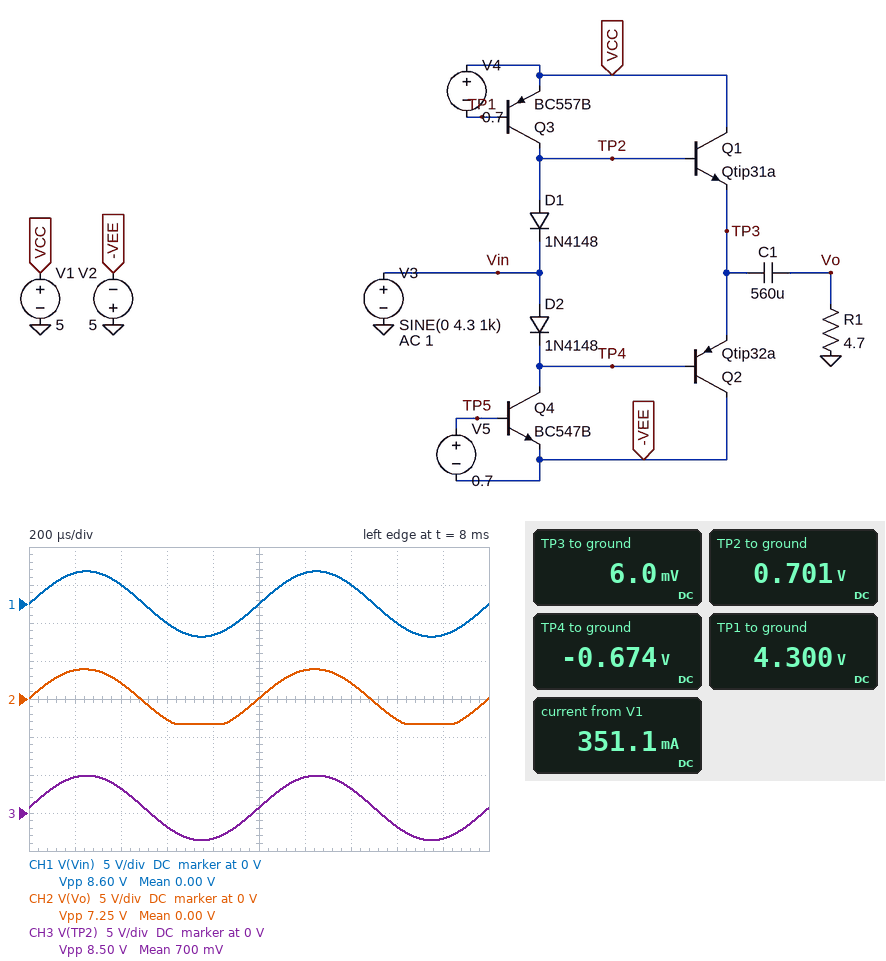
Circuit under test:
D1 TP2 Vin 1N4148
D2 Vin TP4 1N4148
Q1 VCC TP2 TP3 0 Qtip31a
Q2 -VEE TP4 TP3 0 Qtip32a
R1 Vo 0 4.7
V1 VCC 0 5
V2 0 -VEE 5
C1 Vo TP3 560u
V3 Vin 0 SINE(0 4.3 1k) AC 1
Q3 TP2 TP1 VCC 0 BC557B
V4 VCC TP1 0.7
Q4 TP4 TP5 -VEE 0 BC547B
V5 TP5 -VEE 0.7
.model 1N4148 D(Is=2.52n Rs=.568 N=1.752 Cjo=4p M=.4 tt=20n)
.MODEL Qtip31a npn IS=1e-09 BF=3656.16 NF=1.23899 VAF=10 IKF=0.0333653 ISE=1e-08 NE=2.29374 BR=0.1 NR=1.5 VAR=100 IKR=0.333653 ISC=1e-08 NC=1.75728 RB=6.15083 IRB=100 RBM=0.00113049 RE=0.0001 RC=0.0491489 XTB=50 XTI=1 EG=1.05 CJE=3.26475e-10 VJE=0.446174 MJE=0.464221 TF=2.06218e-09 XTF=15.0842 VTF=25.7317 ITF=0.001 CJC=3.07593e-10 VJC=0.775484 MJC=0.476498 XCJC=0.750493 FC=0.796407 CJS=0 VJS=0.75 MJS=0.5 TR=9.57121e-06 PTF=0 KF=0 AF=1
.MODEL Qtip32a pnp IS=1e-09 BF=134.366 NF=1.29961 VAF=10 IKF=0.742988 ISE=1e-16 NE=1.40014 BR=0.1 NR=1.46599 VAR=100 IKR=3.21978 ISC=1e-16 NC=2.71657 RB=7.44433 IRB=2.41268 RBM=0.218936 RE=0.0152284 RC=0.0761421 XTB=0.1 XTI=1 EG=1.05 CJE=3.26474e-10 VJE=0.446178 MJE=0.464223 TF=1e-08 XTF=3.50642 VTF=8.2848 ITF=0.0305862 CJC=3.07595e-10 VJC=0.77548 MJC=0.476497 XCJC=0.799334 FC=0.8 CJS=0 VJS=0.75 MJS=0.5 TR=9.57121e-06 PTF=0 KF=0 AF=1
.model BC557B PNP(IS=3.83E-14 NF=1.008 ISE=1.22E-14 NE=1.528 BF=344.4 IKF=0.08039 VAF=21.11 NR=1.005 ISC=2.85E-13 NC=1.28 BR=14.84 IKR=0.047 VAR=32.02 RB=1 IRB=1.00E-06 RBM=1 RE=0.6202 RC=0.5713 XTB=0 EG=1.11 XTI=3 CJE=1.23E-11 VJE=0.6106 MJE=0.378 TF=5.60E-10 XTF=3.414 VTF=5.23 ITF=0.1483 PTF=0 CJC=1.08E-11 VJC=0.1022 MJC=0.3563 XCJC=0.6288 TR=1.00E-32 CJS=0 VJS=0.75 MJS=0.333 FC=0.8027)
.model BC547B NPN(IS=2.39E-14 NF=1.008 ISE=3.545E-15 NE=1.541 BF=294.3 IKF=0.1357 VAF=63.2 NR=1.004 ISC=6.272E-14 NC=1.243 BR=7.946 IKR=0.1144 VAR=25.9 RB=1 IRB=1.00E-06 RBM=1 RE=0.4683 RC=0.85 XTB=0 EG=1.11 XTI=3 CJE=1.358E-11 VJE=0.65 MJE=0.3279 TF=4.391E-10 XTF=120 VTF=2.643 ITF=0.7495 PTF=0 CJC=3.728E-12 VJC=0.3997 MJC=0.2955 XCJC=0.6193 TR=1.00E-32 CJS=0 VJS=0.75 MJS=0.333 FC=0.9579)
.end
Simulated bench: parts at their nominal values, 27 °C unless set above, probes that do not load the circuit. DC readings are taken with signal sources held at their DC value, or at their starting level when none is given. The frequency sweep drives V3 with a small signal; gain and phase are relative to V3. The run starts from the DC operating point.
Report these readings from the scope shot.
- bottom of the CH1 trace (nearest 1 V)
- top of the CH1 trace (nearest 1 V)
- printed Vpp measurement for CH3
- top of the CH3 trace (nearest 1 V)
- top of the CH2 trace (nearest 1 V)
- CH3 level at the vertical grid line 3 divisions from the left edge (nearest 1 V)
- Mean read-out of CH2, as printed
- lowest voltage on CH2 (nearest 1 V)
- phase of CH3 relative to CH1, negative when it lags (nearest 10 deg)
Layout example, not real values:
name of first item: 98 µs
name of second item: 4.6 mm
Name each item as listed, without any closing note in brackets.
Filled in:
bottom of the CH1 trace: -4 V
top of the CH1 trace: 4 V
printed Vpp measurement for CH3: 8.50 V
top of the CH3 trace: 5 V
top of the CH2 trace: 4 V
CH3 level at the vertical grid line 3 divisions from the left edge: -2 V
Mean read-out of CH2, as printed: 0.00 V
lowest voltage on CH2: -3 V
phase of CH3 relative to CH1, negative when it lags: 0 deg
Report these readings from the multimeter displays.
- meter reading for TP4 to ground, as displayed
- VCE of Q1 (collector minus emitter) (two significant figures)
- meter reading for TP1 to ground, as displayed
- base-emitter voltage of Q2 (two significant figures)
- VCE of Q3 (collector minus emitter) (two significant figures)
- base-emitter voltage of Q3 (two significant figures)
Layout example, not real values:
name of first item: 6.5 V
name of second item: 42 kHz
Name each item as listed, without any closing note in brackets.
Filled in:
meter reading for TP4 to ground, as displayed: -0.674 V
VCE of Q1 (collector minus emitter): 5.0 V
meter reading for TP1 to ground, as displayed: 4.300 V
base-emitter voltage of Q2: -680 mV
VCE of Q3 (collector minus emitter): -4.3 V
base-emitter voltage of Q3: -700 mV
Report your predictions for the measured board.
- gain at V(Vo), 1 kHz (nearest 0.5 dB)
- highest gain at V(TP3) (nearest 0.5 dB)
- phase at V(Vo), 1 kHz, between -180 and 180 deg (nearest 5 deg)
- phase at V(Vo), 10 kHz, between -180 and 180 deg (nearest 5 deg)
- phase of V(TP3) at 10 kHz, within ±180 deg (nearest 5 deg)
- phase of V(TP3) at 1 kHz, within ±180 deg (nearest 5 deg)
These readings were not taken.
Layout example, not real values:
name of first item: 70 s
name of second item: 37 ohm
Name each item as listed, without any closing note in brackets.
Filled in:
gain at V(Vo), 1 kHz: -0.5 dB
highest gain at V(TP3): 0 dB
phase at V(Vo), 1 kHz, between -180 and 180 deg: 5 deg
phase at V(Vo), 10 kHz, between -180 and 180 deg: 0 deg
phase of V(TP3) at 10 kHz, within ±180 deg: 0 deg
phase of V(TP3) at 1 kHz, within ±180 deg: 0 deg
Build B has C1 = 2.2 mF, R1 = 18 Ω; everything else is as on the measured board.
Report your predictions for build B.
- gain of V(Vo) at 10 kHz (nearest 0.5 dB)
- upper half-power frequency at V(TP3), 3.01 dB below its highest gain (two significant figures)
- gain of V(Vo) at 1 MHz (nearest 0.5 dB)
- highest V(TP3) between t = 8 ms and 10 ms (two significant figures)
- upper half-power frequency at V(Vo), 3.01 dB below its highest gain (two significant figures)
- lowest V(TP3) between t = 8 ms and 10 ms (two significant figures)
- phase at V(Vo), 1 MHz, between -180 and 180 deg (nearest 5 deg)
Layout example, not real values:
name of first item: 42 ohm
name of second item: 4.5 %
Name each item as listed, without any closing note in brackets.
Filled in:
gain of V(Vo) at 10 kHz: 0 dB
upper half-power frequency at V(TP3), 3.01 dB below its highest gain: 100 MHz
gain of V(Vo) at 1 MHz: -0.5 dB
highest V(TP3) between t = 8 ms and 10 ms: 4.2 V
upper half-power frequency at V(Vo), 3.01 dB below its highest gain: 110 MHz
lowest V(TP3) between t = 8 ms and 10 ms: -4.2 V
phase at V(Vo), 1 MHz, between -180 and 180 deg: -5 deg
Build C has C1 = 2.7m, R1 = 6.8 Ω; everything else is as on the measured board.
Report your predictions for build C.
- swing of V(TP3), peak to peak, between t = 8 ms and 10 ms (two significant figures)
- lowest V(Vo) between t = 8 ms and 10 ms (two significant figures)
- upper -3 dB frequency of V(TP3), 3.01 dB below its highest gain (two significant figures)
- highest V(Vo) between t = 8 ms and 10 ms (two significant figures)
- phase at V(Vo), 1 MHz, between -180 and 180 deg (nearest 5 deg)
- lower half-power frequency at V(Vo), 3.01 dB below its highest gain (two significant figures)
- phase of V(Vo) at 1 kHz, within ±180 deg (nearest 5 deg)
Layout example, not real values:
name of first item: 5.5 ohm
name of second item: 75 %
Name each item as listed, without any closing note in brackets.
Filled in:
swing of V(TP3), peak to peak, between t = 8 ms and 10 ms: 8.2 V
lowest V(Vo) between t = 8 ms and 10 ms: -4.1 V
upper -3 dB frequency of V(TP3), 3.01 dB below its highest gain: 3.0 MHz
highest V(Vo) between t = 8 ms and 10 ms: 4.1 V
phase at V(Vo), 1 MHz, between -180 and 180 deg: -10 deg
lower half-power frequency at V(Vo), 3.01 dB below its highest gain: 8.5 Hz
phase of V(Vo) at 1 kHz, within ±180 deg: 0 deg
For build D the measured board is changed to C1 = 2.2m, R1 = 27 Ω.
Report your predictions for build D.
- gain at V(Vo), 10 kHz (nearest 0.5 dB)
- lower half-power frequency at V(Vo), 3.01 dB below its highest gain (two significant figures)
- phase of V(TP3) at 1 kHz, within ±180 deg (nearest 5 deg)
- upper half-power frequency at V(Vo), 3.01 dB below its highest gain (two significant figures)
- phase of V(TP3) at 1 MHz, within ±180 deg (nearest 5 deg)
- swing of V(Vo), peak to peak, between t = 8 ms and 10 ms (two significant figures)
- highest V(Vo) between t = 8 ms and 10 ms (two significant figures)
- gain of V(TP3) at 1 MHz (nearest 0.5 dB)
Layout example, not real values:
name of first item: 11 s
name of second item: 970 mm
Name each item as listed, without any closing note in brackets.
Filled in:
gain at V(Vo), 10 kHz: 0 dB
lower half-power frequency at V(Vo), 3.01 dB below its highest gain: 2.7 Hz
phase of V(TP3) at 1 kHz, within ±180 deg: 0 deg
upper half-power frequency at V(Vo), 3.01 dB below its highest gain: 140 MHz
phase of V(TP3) at 1 MHz, within ±180 deg: -5 deg
swing of V(Vo), peak to peak, between t = 8 ms and 10 ms: 8.5 V
highest V(Vo) between t = 8 ms and 10 ms: 4.2 V
gain of V(TP3) at 1 MHz: -0.5 dB
